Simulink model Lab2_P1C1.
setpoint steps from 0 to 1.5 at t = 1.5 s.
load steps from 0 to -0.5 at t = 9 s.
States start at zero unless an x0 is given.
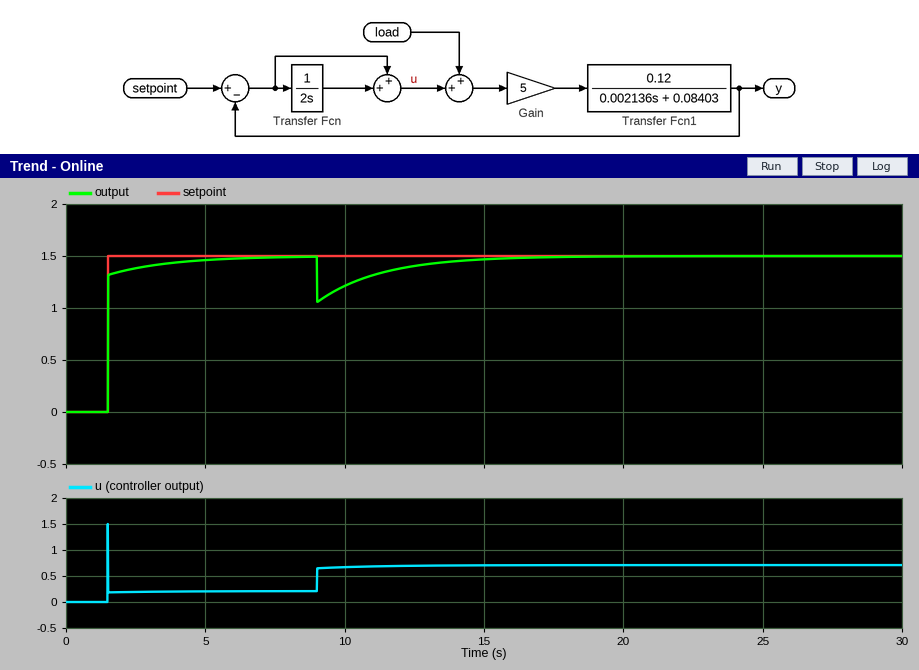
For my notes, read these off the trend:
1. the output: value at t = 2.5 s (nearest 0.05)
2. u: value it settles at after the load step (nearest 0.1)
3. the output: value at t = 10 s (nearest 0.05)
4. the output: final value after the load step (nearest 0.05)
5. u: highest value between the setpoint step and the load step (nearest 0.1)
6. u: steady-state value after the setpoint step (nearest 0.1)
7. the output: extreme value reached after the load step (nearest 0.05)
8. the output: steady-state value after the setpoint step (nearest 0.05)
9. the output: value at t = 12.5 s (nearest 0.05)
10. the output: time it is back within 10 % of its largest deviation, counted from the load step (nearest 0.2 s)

1.40
0.7
1.20
1.50
1.5
0.2
1.05
1.50
1.40
5.4 s
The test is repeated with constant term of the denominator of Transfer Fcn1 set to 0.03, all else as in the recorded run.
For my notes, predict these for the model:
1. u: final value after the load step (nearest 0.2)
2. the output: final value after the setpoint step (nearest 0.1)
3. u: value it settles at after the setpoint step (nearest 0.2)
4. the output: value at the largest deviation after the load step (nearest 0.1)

0.6
1.5
0.0
1.0
